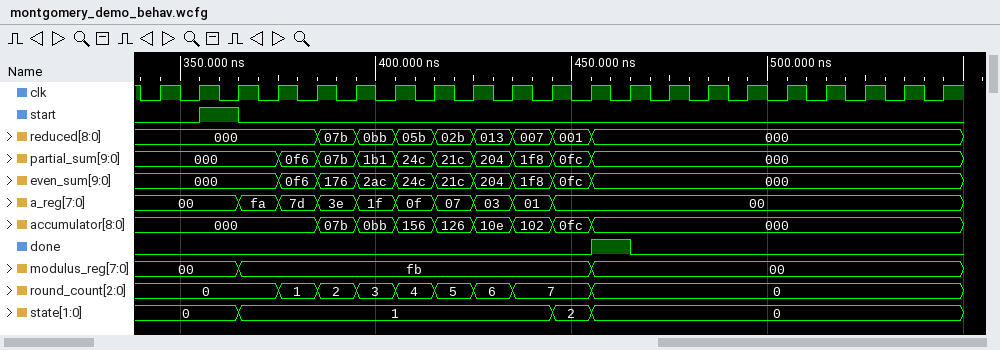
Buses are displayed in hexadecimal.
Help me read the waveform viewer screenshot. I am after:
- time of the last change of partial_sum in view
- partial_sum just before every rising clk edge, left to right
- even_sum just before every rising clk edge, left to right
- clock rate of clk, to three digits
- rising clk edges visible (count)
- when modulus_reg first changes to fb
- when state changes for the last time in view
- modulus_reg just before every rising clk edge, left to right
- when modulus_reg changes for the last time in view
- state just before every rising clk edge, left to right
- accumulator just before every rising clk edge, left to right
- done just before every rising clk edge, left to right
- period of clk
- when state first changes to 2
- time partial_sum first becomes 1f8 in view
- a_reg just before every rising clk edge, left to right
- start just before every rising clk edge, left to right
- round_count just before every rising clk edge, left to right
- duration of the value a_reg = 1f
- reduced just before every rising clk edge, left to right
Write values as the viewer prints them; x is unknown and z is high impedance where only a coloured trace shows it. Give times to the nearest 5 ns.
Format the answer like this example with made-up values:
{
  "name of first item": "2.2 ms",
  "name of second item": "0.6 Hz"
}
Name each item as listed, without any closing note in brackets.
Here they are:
{
  "time of the last change of partial_sum in view": "455 ns",
  "partial_sum just before every rising clk edge, left to right": "000, 000, 000, 000, 0f6, 07b, 1b1, 24c, 21c, 204, 1f8, 0fc, 000, 000, 000, 000, 000, 000, 000, 000, 000",
  "even_sum just before every rising clk edge, left to right": "000, 000, 000, 000, 0f6, 176, 2ac, 24c, 21c, 204, 1f8, 0fc, 000, 000, 000, 000, 000, 000, 000, 000, 000",
  "clock rate of clk, to three digits": "100 MHz",
  "rising clk edges visible": "21",
  "when modulus_reg first changes to fb": "365 ns",
  "when state changes for the last time in view": "455 ns",
  "modulus_reg just before every rising clk edge, left to right": "00, 00, 00, fb, fb, fb, fb, fb, fb, fb, fb, fb, 00, 00, 00, 00, 00, 00, 00, 00, 00",
  "when modulus_reg changes for the last time in view": "455 ns",
  "state just before every rising clk edge, left to right": "0, 0, 0, 1, 1, 1, 1, 1, 1, 1, 1, 2, 0, 0, 0, 0, 0, 0, 0, 0, 0",
  "accumulator just before every rising clk edge, left to right": "000, 000, 000, 000, 000, 07b, 0bb, 156, 126, 10e, 102, 0fc, 000, 000, 000, 000, 000, 000, 000, 000, 000",
  "done just before every rising clk edge, left to right": "0 0 0 0 0 0 0 0 0 0 0 0 1 0 0 0 0 0 0 0 0",
  "period of clk": "10 ns",
  "when state first changes to 2": "445 ns",
  "time partial_sum first becomes 1f8 in view": "435 ns",
  "a_reg just before every rising clk edge, left to right": "00, 00, 00, fa, 7d, 3e, 1f, 0f, 07, 03, 01, 00, 00, 00, 00, 00, 00, 00, 00, 00, 00",
  "start just before every rising clk edge, left to right": "0 0 1 0 0 0 0 0 0 0 0 0 0 0 0 0 0 0 0 0 0",
  "round_count just before every rising clk edge, left to right": "0, 0, 0, 0, 1, 2, 3, 4, 5, 6, 7, 7, 0, 0, 0, 0, 0, 0, 0, 0, 0",
  "duration of the value a_reg = 1f": "10 ns",
  "reduced just before every rising clk edge, left to right": "000, 000, 000, 000, 000, 07b, 0bb, 05b, 02b, 013, 007, 001, 000, 000, 000, 000, 000, 000, 000, 000, 000"
}
